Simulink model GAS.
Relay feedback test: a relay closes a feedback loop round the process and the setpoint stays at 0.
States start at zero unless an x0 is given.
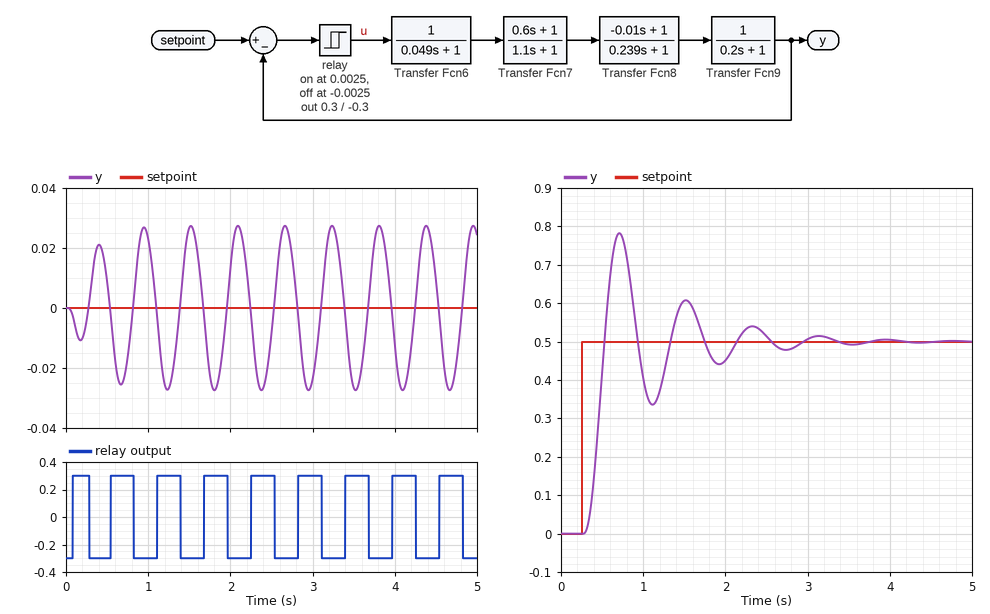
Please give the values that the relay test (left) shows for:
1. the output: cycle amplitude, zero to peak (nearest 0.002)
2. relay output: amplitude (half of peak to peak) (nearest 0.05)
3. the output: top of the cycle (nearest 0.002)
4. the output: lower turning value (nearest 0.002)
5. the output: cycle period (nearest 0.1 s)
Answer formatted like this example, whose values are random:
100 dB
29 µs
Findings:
0.028
0.30
0.028
-0.028
0.6 s
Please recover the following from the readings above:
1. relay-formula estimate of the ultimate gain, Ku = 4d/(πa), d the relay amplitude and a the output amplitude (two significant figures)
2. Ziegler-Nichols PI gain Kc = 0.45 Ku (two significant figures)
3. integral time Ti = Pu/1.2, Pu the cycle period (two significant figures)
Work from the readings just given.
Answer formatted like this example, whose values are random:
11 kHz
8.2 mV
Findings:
14
6.3
0.50 s
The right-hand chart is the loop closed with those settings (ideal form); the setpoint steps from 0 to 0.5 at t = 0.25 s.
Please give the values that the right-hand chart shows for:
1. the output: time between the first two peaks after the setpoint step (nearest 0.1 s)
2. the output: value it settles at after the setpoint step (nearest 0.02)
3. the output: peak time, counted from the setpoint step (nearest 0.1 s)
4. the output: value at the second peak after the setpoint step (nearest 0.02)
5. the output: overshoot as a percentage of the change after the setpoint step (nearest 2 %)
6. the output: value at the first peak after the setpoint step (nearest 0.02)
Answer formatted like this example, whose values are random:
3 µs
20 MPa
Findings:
0.8 s
0.50
0.5 s
0.60
56 %
0.78
